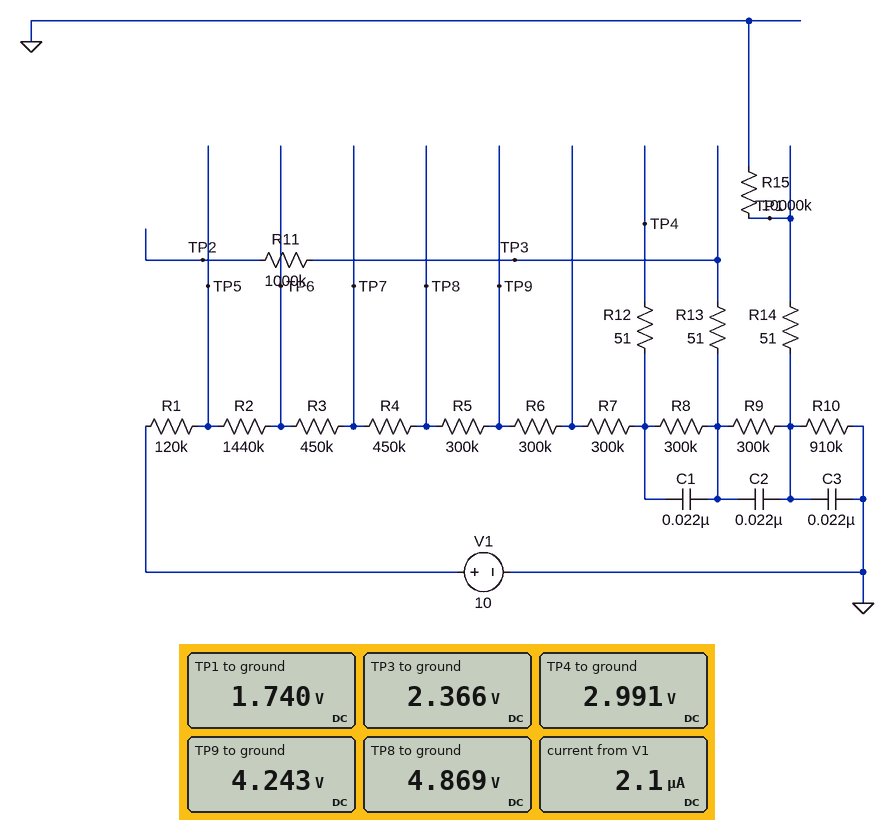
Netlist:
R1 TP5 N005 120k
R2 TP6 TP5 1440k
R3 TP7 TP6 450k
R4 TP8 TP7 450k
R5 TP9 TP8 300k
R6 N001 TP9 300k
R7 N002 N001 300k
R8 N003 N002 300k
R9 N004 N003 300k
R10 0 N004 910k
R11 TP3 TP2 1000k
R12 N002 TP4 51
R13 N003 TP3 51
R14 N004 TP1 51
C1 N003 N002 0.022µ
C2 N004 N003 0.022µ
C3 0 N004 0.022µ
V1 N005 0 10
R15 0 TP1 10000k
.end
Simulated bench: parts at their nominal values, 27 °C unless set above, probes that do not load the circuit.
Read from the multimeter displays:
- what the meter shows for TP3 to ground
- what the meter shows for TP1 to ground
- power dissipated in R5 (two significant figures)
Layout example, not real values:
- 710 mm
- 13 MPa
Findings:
- 2.366 V
- 1.740 V
- 1.3 µW
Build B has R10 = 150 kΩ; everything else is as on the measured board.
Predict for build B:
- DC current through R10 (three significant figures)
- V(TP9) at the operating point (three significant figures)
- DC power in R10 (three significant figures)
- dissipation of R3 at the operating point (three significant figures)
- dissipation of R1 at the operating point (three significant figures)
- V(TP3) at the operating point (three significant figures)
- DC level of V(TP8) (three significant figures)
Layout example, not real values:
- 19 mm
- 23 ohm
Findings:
- 2.40 µA
- 3.28 V
- 863 nW
- 2.67 µW
- 711 nW
- 1.09 V
- 4.01 V
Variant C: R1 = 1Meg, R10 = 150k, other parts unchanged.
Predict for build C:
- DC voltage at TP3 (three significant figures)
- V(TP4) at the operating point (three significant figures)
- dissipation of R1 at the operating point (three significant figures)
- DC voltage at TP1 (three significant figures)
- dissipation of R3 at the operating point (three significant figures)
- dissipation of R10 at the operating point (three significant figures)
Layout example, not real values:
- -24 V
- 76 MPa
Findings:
- 898 mV
- 1.50 V
- 4.02 µW
- 296 mV
- 1.81 µW
- 585 nW
